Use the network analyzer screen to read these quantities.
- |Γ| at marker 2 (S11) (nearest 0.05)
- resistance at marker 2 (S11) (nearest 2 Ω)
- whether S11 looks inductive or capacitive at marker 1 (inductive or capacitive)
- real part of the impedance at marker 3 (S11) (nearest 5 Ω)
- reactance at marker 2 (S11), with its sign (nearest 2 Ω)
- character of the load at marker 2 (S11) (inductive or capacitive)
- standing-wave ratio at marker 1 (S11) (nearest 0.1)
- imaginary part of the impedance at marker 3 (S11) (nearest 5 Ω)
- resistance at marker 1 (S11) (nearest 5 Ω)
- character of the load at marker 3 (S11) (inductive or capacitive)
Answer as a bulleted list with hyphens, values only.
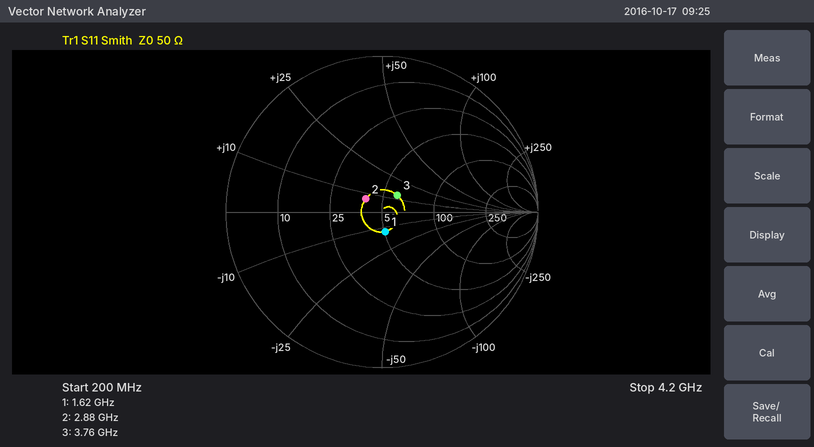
- 0.15
- 40 Ω
- capacitive
- 60 Ω
- +6 Ω
- inductive
- 1.3
- +15 Ω
- 50 Ω
- inductive
